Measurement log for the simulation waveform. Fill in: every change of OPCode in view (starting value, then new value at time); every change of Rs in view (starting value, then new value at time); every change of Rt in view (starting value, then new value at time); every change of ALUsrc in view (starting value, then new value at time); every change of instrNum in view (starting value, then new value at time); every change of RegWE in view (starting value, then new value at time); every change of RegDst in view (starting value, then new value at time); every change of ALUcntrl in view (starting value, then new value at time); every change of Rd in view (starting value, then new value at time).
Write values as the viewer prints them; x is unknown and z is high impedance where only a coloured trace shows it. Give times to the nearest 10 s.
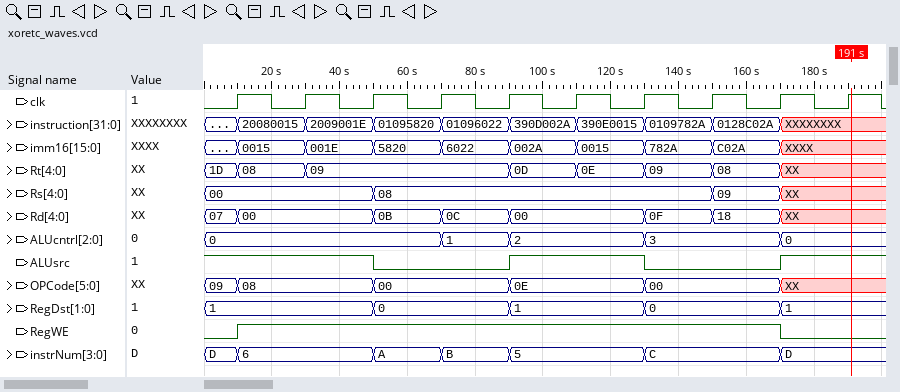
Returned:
09, 08 at 10 s, 00 at 50 s, 0E at 90 s, 00 at 130 s, XX at 170 s
00, 08 at 50 s, 09 at 150 s, XX at 170 s
1D, 08 at 10 s, 09 at 30 s, 0D at 90 s, 0E at 110 s, 09 at 130 s, 08 at 150 s, XX at 170 s
1, 0 at 50 s, 1 at 90 s, 0 at 130 s, 1 at 170 s
D, 6 at 10 s, A at 50 s, B at 70 s, 5 at 90 s, C at 130 s, D at 170 s
0, 1 at 10 s, 0 at 170 s
1, 0 at 50 s, 1 at 90 s, 0 at 130 s, 1 at 170 s
0, 1 at 70 s, 2 at 90 s, 3 at 130 s, 0 at 170 s
07, 00 at 10 s, 0B at 50 s, 0C at 70 s, 00 at 90 s, 0F at 130 s, 18 at 150 s, XX at 170 s
